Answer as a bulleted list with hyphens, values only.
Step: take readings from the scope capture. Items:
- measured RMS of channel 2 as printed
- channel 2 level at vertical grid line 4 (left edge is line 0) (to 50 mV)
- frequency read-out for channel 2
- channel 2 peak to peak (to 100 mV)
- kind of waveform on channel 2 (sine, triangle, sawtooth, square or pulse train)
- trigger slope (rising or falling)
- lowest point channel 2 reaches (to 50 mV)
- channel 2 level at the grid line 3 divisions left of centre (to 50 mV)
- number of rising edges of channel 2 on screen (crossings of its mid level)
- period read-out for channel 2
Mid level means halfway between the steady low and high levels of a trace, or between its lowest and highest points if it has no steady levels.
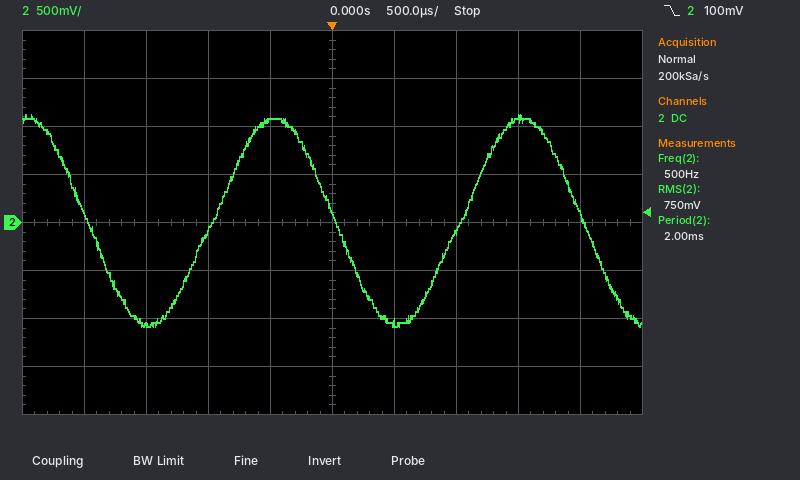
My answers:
- 750 mV
- 1.05 V
- 500 Hz
- 2.20 V
- sine
- falling
- -1.10 V
- -1.05 V
- 2
- 2.00 ms
